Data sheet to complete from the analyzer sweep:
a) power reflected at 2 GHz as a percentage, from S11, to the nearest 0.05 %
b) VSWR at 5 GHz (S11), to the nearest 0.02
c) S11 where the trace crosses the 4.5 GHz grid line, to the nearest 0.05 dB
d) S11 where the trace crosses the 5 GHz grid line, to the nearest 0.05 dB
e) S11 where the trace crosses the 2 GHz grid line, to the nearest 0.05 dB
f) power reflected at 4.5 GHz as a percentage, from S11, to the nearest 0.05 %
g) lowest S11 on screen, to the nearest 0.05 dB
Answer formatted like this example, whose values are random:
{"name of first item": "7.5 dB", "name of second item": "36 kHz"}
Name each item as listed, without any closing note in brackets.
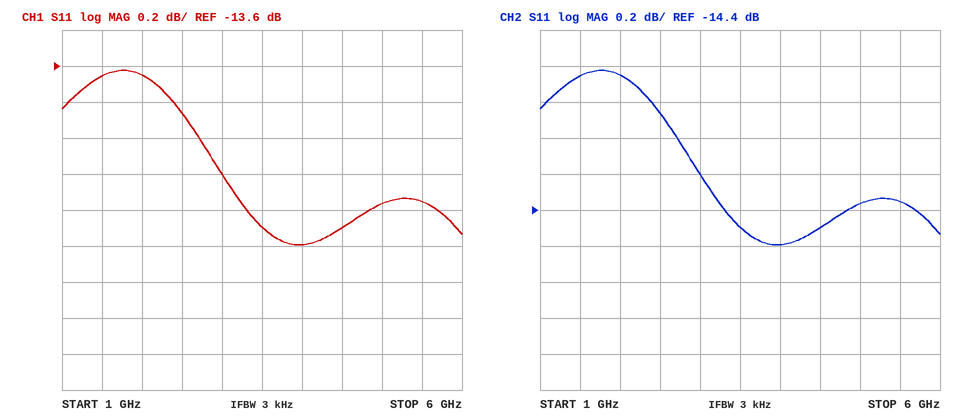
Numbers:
{"power reflected at 2 GHz as a percentage, from S11, to the nearest 0.05 %": "4.30 %", "VSWR at 5 GHz (S11), to the nearest 0.02": "1.48", "S11 where the trace crosses the 4.5 GHz grid line, to the nearest 0.05 dB": "-14.50 dB", "S11 where the trace crosses the 5 GHz grid line, to the nearest 0.05 dB": "-14.35 dB", "S11 where the trace crosses the 2 GHz grid line, to the nearest 0.05 dB": "-13.65 dB", "power reflected at 4.5 GHz as a percentage, from S11, to the nearest 0.05 %": "3.55 %", "lowest S11 on screen, to the nearest 0.05 dB": "-14.60 dB"}
